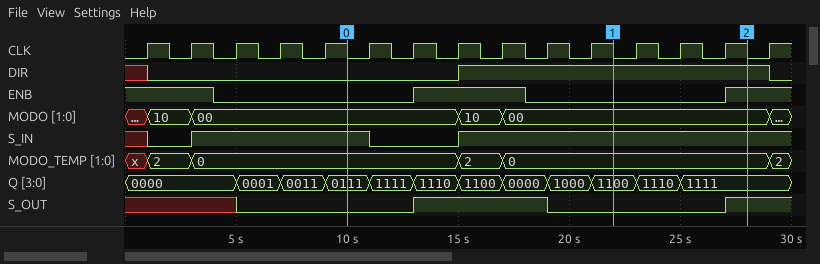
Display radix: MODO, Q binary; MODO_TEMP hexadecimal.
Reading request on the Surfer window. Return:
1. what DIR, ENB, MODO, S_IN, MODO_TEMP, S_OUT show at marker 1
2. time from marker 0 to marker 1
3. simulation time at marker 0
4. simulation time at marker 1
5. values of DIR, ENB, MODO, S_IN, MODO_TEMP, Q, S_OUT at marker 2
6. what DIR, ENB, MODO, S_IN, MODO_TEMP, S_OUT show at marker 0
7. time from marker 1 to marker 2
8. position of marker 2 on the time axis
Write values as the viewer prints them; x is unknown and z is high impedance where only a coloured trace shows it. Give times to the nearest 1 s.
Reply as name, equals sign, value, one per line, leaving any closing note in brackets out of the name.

what DIR, ENB, MODO, S_IN, MODO_TEMP, S_OUT show at marker 1 = DIR=1, ENB=0, MODO=00, S_IN=1, MODO_TEMP=0, S_OUT=0
time from marker 0 to marker 1 = 12 s
simulation time at marker 0 = 10 s
simulation time at marker 1 = 22 s
values of DIR, ENB, MODO, S_IN, MODO_TEMP, Q, S_OUT at marker 2 = DIR=1, ENB=1, MODO=00, S_IN=1, MODO_TEMP=0, Q=1111, S_OUT=1
what DIR, ENB, MODO, S_IN, MODO_TEMP, S_OUT show at marker 0 = DIR=0, ENB=0, MODO=00, S_IN=1, MODO_TEMP=0, S_OUT=0
time from marker 1 to marker 2 = 6 s
position of marker 2 on the time axis = 28 s
